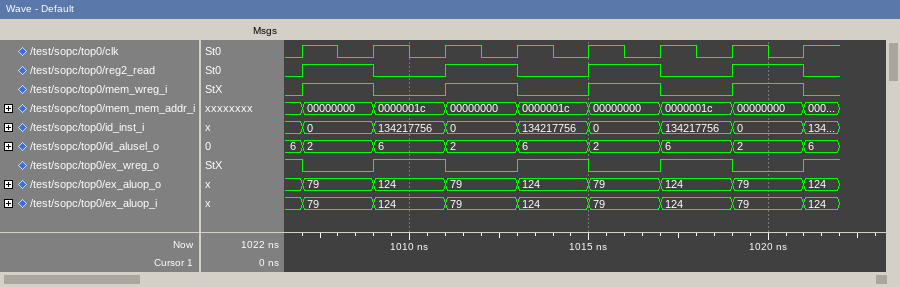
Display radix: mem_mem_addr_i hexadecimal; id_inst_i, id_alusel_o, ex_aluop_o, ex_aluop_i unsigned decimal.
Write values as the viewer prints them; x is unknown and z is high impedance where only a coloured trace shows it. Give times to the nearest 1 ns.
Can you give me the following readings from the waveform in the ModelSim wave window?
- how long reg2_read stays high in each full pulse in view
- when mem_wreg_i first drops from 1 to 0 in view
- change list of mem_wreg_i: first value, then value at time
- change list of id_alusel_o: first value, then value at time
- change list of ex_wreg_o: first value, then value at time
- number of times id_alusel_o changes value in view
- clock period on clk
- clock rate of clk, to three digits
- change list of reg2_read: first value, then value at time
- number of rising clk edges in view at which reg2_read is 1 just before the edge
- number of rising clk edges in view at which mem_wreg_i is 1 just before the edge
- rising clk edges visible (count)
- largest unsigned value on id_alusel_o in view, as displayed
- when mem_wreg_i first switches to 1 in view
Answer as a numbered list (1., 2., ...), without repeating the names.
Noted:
1. 2 ns, 2 ns, 2 ns, 2 ns
2. 1009 ns
3. 0, 1 at 1007 ns, 0 at 1009 ns, 1 at 1011 ns, 0 at 1013 ns, 1 at 1015 ns, 0 at 1017 ns, 1 at 1019 ns, 0 at 1021 ns
4. 6, 2 at 1007 ns, 6 at 1009 ns, 2 at 1011 ns, 6 at 1013 ns, 2 at 1015 ns, 6 at 1017 ns, 2 at 1019 ns, 6 at 1021 ns
5. 1, 0 at 1007 ns, 1 at 1009 ns, 0 at 1011 ns, 1 at 1013 ns, 0 at 1015 ns, 1 at 1017 ns, 0 at 1019 ns, 1 at 1021 ns
6. 8
7. 2 ns
8. 500 MHz
9. 0, 1 at 1007 ns, 0 at 1009 ns, 1 at 1011 ns, 0 at 1013 ns, 1 at 1015 ns, 0 at 1017 ns, 1 at 1019 ns, 0 at 1021 ns
10. 4
11. 4
12. 8
13. 6
14. 1007 ns
